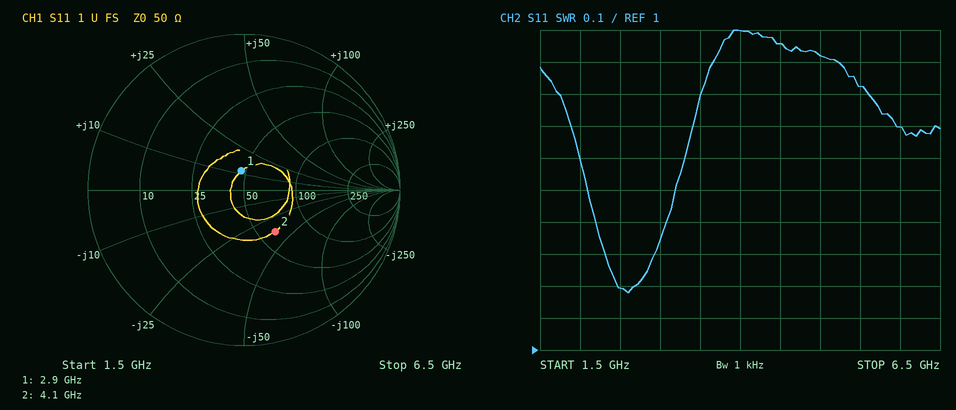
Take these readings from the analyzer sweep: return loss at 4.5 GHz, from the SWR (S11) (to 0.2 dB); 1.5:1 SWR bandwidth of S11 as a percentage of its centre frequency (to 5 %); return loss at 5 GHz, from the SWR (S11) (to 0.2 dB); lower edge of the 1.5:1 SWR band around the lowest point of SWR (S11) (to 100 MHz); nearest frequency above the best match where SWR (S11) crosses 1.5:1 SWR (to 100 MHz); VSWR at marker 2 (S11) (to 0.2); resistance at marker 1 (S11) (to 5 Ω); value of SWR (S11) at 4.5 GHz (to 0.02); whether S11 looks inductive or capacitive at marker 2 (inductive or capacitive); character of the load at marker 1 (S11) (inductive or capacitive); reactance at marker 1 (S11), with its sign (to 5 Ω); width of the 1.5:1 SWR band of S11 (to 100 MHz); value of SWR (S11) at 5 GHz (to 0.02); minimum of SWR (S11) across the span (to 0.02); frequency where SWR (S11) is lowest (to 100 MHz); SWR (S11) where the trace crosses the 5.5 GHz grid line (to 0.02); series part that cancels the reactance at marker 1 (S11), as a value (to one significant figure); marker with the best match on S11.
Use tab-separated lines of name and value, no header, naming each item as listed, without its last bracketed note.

return loss at 4.5 GHz, from the SWR (S11)	9.8 dB
1.5:1 SWR bandwidth of S11 as a percentage of its centre frequency	40 %
return loss at 5 GHz, from the SWR (S11)	10.0 dB
lower edge of the 1.5:1 SWR band around the lowest point of SWR (S11)	2.1 GHz
nearest frequency above the best match where SWR (S11) crosses 1.5:1 SWR	3.2 GHz
VSWR at marker 2 (S11)	2.0
resistance at marker 1 (S11)	45 Ω
value of SWR (S11) at 4.5 GHz	1.96
whether S11 looks inductive or capacitive at marker 2	capacitive
character of the load at marker 1 (S11)	inductive
reactance at marker 1 (S11), with its sign	+10 Ω
width of the 1.5:1 SWR band of S11	1.1 GHz
value of SWR (S11) at 5 GHz	1.92
minimum of SWR (S11) across the span	1.18
frequency where SWR (S11) is lowest	2.6 GHz
SWR (S11) where the trace crosses the 5.5 GHz grid line	1.82
series part that cancels the reactance at marker 1 (S11), as a value	5 pF
marker with the best match on S11	marker 1
